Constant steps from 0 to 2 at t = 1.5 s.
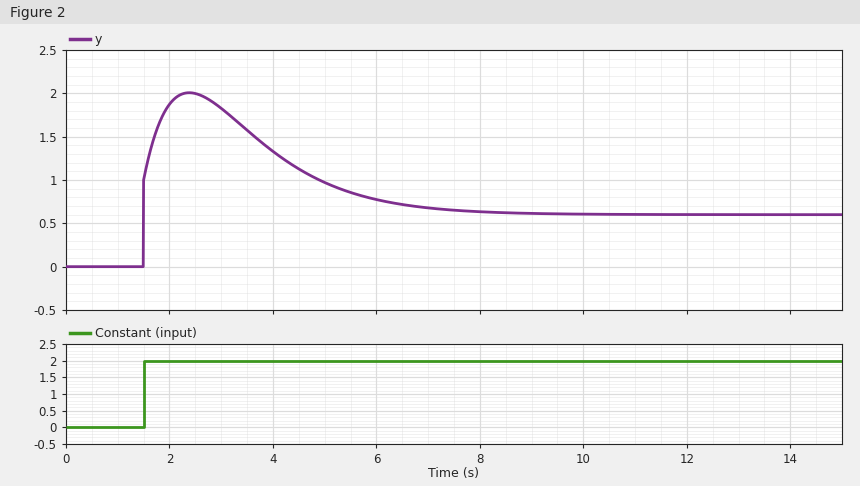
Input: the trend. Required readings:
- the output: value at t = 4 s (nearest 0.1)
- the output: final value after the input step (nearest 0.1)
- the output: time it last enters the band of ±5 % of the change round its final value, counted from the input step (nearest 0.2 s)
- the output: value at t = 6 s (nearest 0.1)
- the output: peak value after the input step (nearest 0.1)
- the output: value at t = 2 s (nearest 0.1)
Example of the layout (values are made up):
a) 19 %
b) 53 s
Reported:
a) 1.3
b) 0.6
c) 6.6 s
d) 0.8
e) 2.0
f) 1.9
